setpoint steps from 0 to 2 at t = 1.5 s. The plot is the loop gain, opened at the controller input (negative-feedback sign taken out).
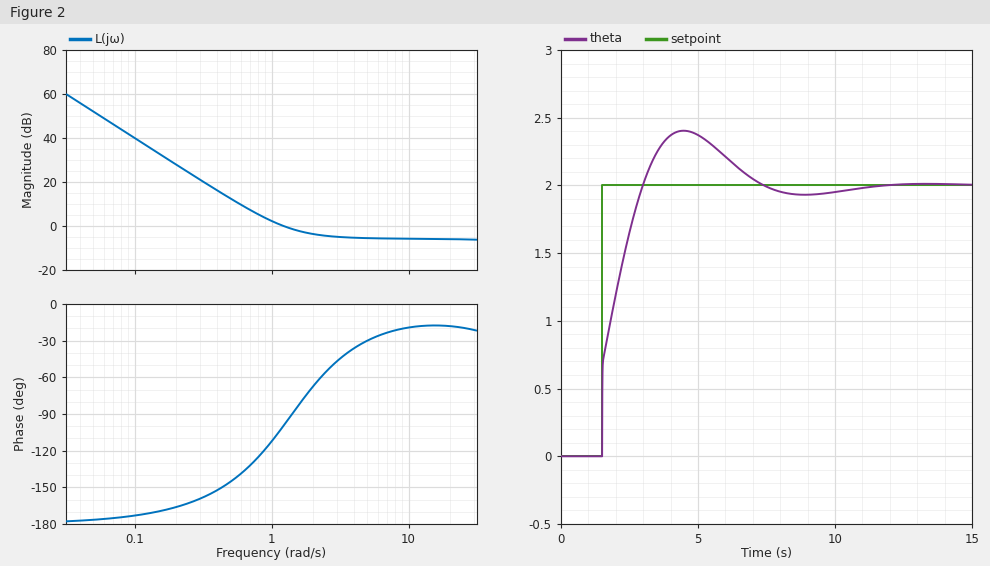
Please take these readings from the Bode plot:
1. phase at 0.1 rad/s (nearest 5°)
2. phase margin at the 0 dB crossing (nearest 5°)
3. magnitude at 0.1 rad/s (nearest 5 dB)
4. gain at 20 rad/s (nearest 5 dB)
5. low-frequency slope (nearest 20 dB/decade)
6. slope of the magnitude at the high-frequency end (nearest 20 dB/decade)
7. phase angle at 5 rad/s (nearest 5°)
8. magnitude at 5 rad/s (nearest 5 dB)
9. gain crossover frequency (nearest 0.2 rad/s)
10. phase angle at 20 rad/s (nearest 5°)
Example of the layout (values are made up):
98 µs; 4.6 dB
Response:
-175°; 80°; 40 dB; -5 dB; -40 dB/decade; 0 dB/decade; -30°; -5 dB; 1.2 rad/s; -20°
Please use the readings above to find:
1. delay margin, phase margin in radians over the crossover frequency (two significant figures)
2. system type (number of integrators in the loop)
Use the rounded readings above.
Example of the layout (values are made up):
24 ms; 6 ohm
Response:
1.2 s; 2
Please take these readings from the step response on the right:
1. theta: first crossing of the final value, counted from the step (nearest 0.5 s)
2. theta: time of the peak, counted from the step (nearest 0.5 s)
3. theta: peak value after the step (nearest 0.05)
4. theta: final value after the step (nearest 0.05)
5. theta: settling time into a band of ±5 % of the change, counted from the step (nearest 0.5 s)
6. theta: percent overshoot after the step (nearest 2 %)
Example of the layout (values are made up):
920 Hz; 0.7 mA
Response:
1.5 s; 3.0 s; 2.40; 2.00; 5.0 s; 20 %
